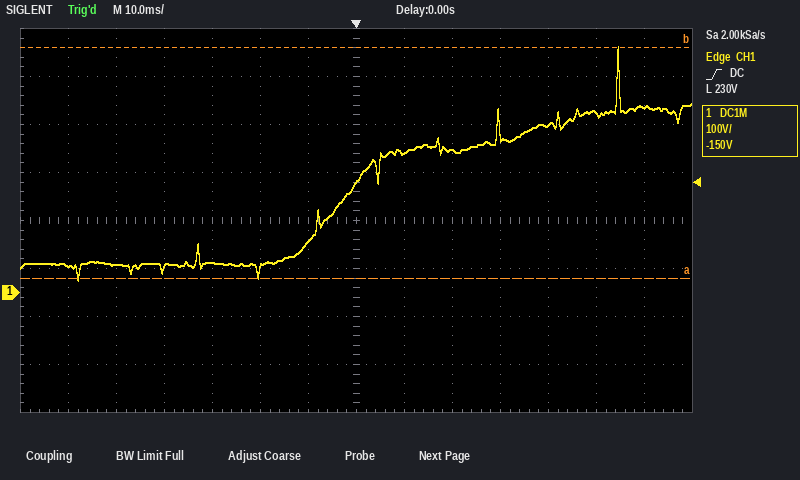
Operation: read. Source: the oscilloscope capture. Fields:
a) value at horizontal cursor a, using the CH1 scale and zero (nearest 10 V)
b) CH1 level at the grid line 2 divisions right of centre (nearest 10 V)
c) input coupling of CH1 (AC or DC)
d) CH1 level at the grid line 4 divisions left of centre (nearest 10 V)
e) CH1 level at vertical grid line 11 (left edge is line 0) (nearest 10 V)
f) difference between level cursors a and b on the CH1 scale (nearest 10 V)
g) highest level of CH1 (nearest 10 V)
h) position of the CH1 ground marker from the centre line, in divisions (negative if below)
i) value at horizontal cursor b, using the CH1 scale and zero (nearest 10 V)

30 V
300 V
DC
50 V
350 V
480 V
510 V
-1.5 div
510 V
